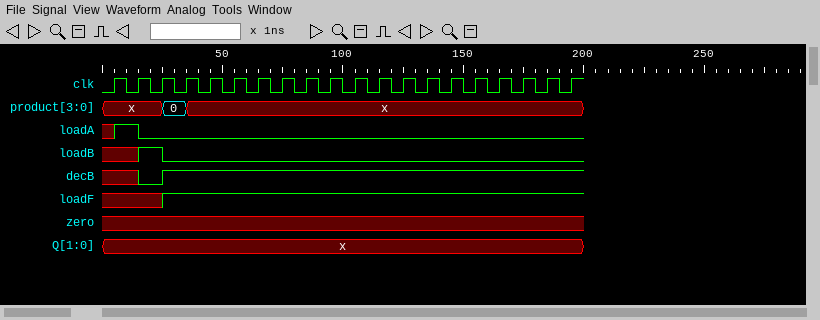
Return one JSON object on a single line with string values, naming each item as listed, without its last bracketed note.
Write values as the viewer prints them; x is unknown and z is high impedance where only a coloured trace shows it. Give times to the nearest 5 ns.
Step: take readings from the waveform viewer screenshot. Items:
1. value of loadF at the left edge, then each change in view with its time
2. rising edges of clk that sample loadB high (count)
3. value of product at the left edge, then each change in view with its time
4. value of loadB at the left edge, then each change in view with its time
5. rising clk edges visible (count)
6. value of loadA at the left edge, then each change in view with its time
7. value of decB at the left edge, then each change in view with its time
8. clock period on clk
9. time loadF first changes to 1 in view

{"value of loadF at the left edge, then each change in view with its time": "x, 1 at 25 ns", "rising edges of clk that sample loadB high": "1", "value of product at the left edge, then each change in view with its time": "x, 0 at 25 ns, x at 35 ns", "value of loadB at the left edge, then each change in view with its time": "x, 1 at 15 ns, 0 at 25 ns", "rising clk edges visible": "20", "value of loadA at the left edge, then each change in view with its time": "x, 1 at 5 ns, 0 at 15 ns", "value of decB at the left edge, then each change in view with its time": "x, 0 at 15 ns, 1 at 25 ns", "clock period on clk": "10 ns", "time loadF first changes to 1 in view": "25 ns"}
